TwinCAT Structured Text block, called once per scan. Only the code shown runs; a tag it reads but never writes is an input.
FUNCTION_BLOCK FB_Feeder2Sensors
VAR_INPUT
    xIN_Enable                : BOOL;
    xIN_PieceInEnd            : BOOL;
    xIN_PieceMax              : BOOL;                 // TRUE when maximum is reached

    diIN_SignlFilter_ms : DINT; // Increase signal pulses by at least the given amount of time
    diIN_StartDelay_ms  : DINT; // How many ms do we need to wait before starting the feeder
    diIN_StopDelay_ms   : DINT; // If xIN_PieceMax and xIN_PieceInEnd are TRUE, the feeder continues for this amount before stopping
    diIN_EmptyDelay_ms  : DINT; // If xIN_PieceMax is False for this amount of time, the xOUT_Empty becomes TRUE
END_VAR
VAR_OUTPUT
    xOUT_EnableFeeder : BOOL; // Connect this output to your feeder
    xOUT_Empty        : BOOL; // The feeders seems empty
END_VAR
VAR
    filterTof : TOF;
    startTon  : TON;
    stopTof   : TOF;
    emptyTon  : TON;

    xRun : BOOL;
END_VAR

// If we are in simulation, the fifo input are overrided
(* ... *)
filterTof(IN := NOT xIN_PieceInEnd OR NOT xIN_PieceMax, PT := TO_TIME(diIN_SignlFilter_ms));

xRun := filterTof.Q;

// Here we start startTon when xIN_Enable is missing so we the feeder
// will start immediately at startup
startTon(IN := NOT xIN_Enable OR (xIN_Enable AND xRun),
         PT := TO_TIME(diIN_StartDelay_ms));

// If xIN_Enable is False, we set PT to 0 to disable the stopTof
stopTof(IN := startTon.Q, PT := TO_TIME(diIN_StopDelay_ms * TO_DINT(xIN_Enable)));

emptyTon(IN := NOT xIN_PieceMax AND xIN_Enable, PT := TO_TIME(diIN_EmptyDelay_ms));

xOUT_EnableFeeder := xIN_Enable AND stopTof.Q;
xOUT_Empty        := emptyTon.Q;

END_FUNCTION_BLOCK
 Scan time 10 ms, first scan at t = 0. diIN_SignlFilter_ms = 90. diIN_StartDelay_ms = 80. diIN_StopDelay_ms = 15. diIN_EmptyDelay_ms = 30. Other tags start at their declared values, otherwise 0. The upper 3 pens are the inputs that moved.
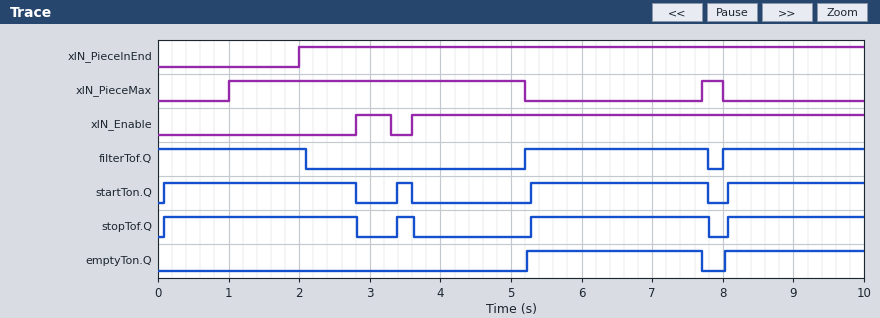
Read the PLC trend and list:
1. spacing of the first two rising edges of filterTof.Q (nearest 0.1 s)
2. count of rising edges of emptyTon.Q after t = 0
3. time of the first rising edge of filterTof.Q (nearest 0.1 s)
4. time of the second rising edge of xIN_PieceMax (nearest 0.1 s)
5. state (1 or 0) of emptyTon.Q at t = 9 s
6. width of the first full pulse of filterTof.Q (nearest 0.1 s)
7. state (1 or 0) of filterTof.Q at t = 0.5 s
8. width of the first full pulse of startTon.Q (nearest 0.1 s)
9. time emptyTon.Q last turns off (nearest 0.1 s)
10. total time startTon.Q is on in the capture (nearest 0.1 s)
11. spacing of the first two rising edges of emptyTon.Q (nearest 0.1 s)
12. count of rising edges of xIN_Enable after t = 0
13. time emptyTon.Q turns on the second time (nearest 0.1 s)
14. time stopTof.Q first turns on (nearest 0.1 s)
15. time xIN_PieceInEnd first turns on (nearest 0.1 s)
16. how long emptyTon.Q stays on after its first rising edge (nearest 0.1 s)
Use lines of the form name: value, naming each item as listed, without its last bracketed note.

spacing of the first two rising edges of filterTof.Q: 2.8 s
count of rising edges of emptyTon.Q after t = 0: 2
time of the first rising edge of filterTof.Q: 5.2 s
time of the second rising edge of xIN_PieceMax: 7.7 s
state (1 or 0) of emptyTon.Q at t = 9 s: 1
width of the first full pulse of filterTof.Q: 2.6 s
state (1 or 0) of filterTof.Q at t = 0.5 s: 1
width of the first full pulse of startTon.Q: 2.7 s
time emptyTon.Q last turns off: 7.7 s
total time startTon.Q is on in the capture: 7.4 s
spacing of the first two rising edges of emptyTon.Q: 2.8 s
count of rising edges of xIN_Enable after t = 0: 2
time emptyTon.Q turns on the second time: 8.0 s
time stopTof.Q first turns on: 0.1 s
time xIN_PieceInEnd first turns on: 2.0 s
how long emptyTon.Q stays on after its first rising edge: 2.5 s
